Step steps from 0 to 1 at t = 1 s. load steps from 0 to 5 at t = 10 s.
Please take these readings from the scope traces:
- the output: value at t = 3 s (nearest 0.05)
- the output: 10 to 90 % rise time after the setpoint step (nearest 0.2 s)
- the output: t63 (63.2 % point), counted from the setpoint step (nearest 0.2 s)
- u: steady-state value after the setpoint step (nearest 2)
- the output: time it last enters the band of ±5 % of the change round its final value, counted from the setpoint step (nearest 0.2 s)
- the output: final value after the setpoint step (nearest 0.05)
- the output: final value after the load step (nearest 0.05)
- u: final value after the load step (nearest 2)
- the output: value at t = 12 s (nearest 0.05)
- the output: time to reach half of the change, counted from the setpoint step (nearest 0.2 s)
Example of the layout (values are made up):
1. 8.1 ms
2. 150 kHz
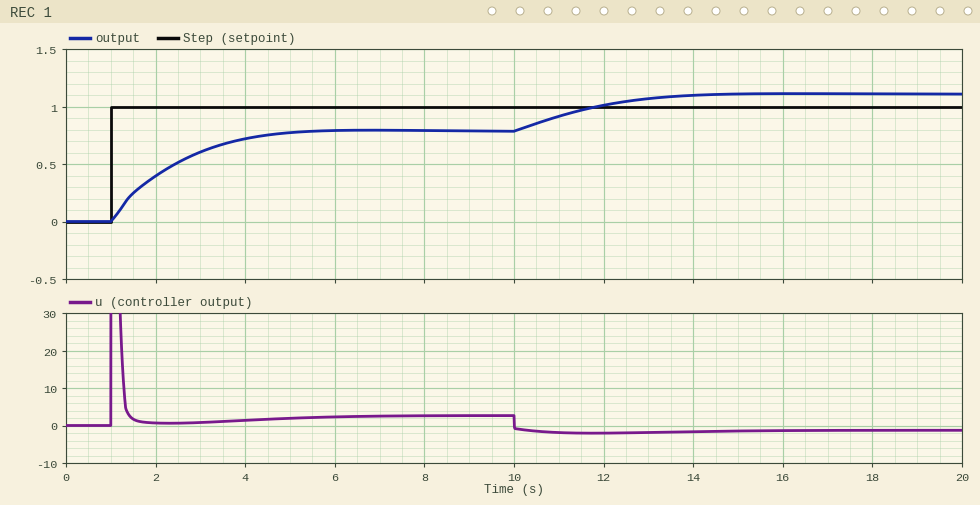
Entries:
1. 0.60
2. 2.6 s
3. 1.4 s
4. 2
5. 3.4 s
6. 0.80
7. 1.10
8. -2
9. 1.00
10. 1.0 s
